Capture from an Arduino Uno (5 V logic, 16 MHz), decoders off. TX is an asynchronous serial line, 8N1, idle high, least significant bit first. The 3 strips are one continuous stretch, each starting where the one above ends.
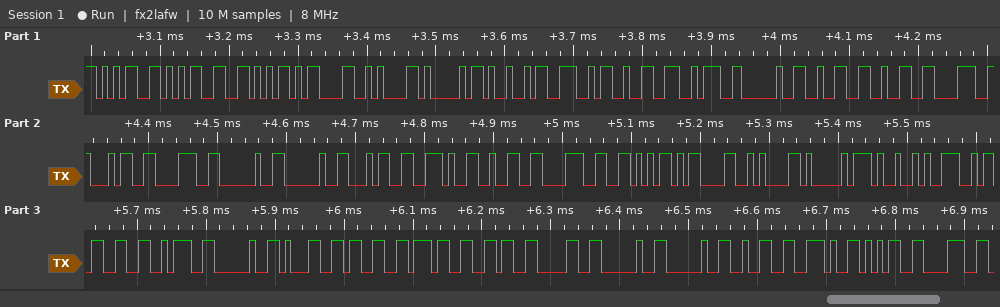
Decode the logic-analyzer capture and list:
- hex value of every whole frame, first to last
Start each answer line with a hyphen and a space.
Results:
- 35 35 56 0D 0A 41 49 4E 32 3A 20 32 32 38 34 38 20 20 34 2E 32 38 56 0D 0A 41 49 4E 33 3A 20 31 33 37 36 30 20 20 32 2E 35 38
